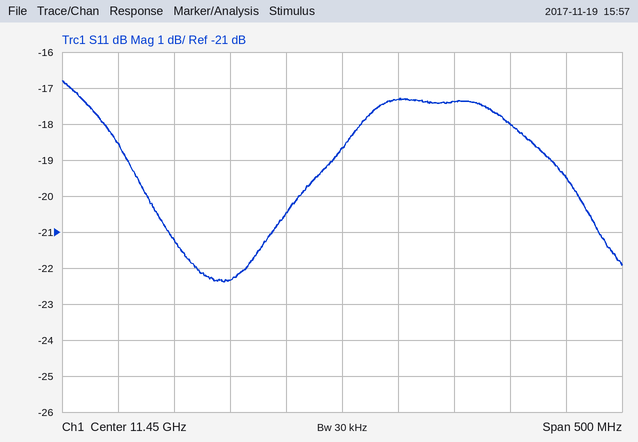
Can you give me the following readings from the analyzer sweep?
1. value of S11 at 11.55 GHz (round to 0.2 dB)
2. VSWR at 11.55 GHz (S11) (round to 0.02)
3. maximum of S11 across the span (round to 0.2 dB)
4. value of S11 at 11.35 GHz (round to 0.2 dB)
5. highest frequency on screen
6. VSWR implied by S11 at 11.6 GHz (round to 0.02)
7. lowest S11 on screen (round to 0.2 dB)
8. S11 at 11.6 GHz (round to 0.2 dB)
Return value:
-17.4 dB
1.32
-16.8 dB
-22.4 dB
11.7 GHz
1.28
-22.4 dB
-18.0 dB
